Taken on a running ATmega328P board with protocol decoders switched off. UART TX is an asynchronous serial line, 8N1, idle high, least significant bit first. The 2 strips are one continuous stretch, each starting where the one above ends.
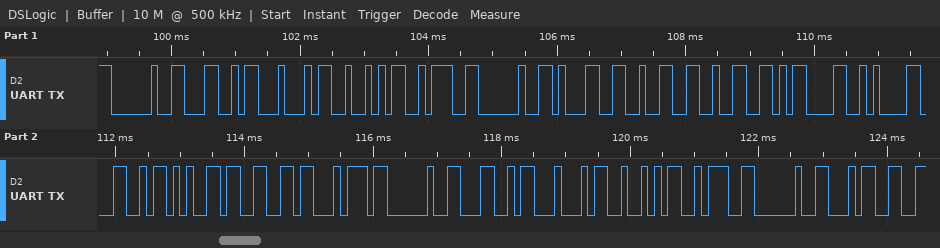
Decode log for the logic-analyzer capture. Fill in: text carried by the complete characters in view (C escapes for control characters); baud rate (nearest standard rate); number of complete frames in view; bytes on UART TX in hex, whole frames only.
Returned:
" LDR: 122\r\nLeft LDR: 4"
9600 baud
22
0x20 0x4C 0x44 0x52 0x3A 0x20 0x31 0x32 0x32 0x0D 0x0A 0x4C 0x65 0x66 0x74 0x20 0x4C 0x44 0x52 0x3A 0x20 0x34
